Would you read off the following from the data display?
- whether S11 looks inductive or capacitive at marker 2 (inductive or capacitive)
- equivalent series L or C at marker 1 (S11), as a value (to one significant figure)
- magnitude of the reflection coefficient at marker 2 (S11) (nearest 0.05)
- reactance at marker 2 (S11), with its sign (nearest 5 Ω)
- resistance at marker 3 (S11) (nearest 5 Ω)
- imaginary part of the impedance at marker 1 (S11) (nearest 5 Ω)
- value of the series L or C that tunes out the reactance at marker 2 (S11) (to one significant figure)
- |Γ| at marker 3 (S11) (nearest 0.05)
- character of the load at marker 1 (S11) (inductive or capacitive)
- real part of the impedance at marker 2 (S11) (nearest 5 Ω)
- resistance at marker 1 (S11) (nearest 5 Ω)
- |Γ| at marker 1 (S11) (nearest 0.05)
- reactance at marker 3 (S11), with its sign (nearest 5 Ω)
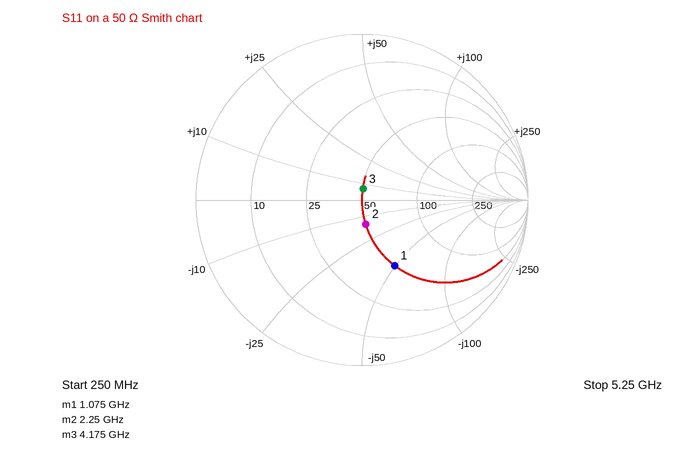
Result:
capacitive
3 pF
0.15
-15 Ω
50 Ω
-50 Ω
1 nH
0.05
capacitive
50 Ω
50 Ω
0.45
+5 Ω
